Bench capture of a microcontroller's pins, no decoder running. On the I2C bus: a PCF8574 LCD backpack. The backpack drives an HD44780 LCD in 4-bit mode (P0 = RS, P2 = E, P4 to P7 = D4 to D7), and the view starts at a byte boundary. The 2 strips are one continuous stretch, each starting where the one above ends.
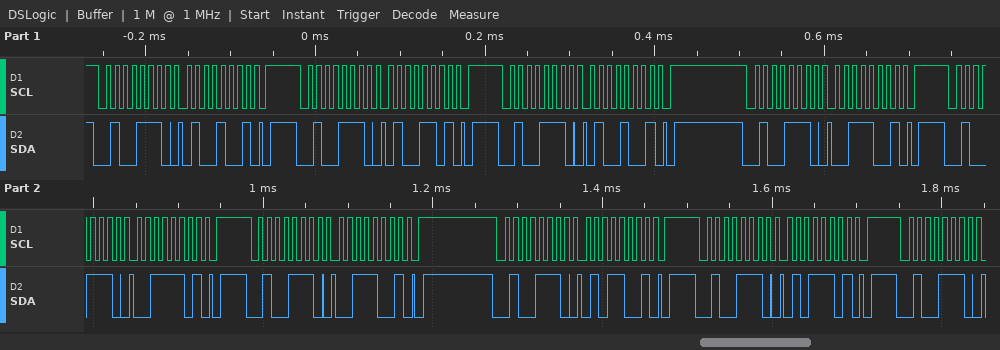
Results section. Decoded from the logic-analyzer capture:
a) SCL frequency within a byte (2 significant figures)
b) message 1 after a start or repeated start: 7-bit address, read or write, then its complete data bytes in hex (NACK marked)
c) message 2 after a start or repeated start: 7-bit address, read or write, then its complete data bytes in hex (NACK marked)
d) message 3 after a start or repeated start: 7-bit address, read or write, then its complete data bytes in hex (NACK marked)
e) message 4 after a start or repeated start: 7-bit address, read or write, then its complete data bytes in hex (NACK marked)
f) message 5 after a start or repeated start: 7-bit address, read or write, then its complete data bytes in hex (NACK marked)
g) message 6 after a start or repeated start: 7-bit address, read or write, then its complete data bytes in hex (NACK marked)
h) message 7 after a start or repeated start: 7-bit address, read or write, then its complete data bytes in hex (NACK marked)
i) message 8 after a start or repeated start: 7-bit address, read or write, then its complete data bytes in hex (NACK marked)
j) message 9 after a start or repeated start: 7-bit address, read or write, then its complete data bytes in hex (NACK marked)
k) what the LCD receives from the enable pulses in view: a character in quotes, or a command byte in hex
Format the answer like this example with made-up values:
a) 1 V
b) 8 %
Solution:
a) 100 kHz
b) 0x27 write: 49
c) 0x27 write: 4D
d) 0x27 write: 49
e) 0x27 write: 39
f) 0x27 write: 3D
g) 0x27 write: 39
h) 0x27 write: 59
i) 0x27 write: 5D
j) 0x27 write
k) 'C'
